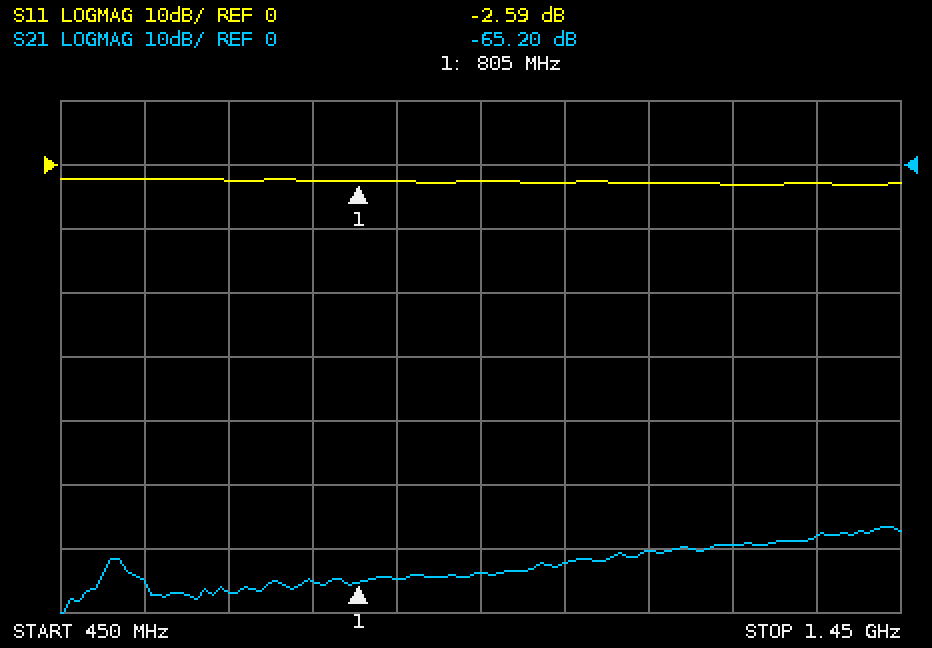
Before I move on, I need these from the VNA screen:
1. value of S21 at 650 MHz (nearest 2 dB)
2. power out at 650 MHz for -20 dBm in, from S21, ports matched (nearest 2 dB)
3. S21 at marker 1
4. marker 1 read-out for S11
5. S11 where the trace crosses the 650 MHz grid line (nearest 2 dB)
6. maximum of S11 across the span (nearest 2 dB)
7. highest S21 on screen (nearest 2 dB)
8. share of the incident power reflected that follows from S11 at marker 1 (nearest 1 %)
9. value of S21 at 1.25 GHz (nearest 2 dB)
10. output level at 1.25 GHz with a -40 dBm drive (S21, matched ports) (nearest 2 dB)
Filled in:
-66 dB
-86 dBm
-65.20 dB
-2.59 dB
-2 dB
-2 dB
-56 dB
55 %
-60 dB
-100 dBm
